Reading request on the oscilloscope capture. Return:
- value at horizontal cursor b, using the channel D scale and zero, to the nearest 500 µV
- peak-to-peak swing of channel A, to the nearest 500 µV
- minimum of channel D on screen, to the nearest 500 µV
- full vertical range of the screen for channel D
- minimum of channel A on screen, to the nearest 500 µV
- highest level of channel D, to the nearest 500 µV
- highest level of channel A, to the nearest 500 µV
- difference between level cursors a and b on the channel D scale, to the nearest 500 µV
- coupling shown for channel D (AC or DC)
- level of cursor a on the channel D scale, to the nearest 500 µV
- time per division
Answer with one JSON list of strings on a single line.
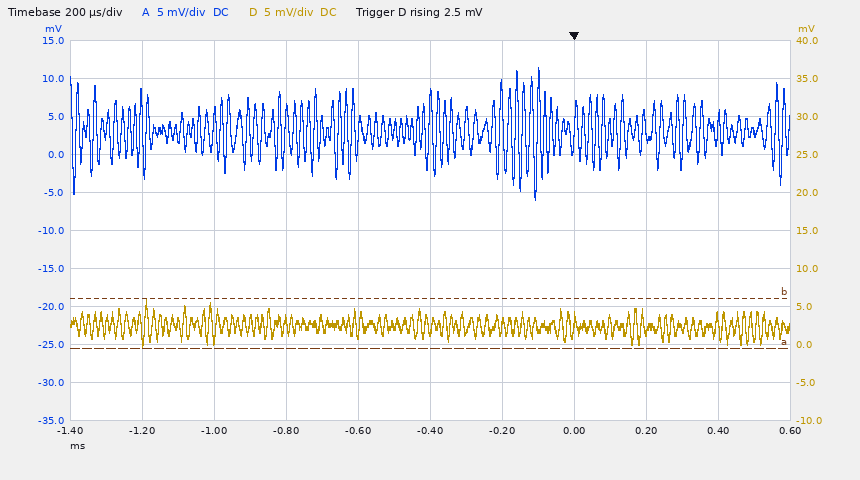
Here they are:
["6.0 mV", "17.5 mV", "-500 µV", "50 mV", "-6.0 mV", "6.0 mV", "11.5 mV", "6.5 mV", "DC", "-500 µV", "200 µs"]
